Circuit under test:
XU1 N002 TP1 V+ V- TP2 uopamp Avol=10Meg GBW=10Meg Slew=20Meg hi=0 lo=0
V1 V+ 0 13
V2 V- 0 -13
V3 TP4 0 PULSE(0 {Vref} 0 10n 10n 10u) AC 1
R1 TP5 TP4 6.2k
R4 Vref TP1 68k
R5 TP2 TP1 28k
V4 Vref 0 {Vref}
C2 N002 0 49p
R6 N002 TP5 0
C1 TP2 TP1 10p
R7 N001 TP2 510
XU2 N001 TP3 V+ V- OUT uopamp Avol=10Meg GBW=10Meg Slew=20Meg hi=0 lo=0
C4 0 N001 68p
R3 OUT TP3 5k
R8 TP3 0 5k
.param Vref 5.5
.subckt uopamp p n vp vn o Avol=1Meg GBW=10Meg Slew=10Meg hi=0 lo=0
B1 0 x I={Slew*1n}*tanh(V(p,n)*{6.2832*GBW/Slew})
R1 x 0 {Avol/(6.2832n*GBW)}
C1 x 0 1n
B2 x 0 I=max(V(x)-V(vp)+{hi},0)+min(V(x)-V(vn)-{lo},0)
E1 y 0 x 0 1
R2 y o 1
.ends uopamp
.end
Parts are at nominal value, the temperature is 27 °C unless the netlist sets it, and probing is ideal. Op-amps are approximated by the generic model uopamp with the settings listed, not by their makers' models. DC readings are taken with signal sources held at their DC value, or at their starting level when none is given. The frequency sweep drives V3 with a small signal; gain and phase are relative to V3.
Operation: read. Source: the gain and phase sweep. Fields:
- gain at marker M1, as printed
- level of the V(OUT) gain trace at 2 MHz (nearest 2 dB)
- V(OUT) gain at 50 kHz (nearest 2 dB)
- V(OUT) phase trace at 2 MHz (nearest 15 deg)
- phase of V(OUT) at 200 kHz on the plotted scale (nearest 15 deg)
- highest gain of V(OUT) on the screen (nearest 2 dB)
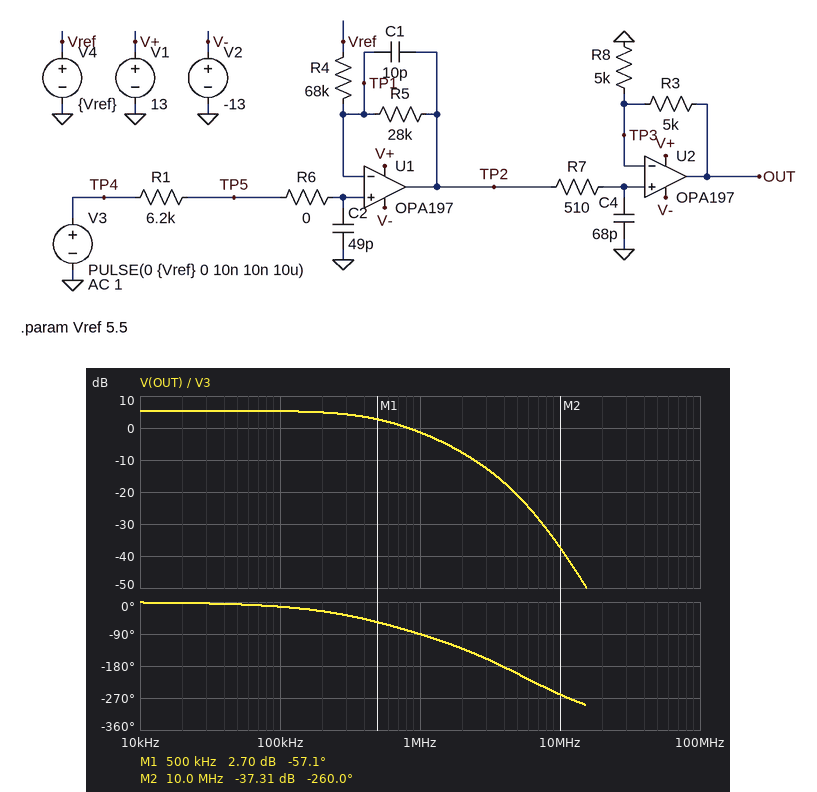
2.70 dB
-8 dB
6 dB
-135 deg
-30 deg
6 dB
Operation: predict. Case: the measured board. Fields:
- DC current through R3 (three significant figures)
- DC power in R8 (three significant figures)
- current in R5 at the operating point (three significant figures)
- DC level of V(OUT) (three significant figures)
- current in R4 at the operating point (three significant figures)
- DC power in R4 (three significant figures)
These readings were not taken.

453 µA
1.03 mW
80.9 µA
-4.53 V
80.9 µA
445 µW
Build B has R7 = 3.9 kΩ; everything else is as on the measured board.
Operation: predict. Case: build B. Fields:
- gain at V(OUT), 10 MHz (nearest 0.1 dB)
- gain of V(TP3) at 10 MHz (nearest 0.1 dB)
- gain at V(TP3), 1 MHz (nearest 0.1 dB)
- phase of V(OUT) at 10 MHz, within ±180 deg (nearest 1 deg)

-54.2 dB
-60.2 dB
-12.9 dB
79 deg
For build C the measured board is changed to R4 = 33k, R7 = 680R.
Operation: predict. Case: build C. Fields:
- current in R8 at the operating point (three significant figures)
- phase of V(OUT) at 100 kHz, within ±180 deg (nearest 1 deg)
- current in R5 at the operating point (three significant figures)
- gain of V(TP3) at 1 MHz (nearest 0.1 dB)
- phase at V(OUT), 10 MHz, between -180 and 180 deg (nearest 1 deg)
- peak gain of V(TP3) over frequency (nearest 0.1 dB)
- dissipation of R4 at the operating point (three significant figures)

933 µA
-16 deg
167 µA
-6.6 dB
94 deg
1.7 dB
917 µW
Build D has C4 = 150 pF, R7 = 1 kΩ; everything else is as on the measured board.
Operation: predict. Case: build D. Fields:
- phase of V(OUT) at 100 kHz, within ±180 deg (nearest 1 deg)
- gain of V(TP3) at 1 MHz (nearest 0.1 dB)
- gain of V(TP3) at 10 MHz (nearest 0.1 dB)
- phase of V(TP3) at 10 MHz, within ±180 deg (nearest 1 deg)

-17 deg
-9.9 dB
-55.3 dB
81 deg
